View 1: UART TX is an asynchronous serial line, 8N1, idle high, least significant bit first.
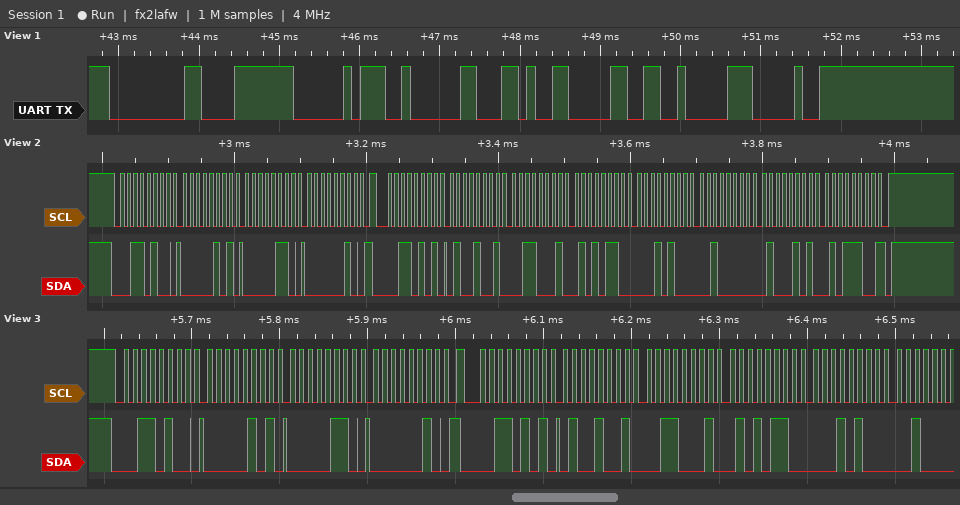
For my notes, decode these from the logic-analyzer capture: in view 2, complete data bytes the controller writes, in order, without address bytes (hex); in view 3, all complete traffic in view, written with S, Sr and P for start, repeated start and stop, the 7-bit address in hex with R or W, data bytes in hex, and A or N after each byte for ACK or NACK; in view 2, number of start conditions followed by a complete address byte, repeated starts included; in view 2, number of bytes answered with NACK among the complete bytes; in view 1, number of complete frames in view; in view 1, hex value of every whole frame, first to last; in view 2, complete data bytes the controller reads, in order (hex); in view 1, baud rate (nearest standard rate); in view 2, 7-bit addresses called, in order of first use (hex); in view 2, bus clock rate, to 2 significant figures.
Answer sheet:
05 06 02
S 1AW A 05 A 06 A 02 A Sr 1AR A 49 A 31 A 56 A 14 A
2
1
8
00 F8 A0 02 2C 30 82 90
49 31 56 14 20 45 5C
9600 baud
0x1A
100 kHz
